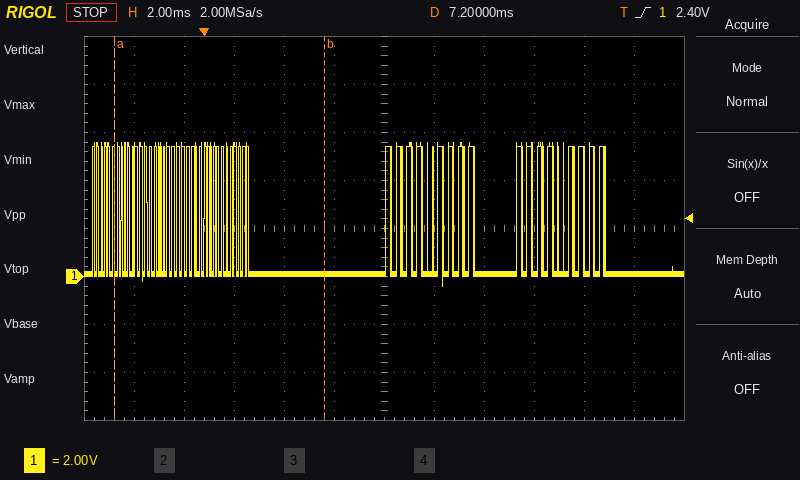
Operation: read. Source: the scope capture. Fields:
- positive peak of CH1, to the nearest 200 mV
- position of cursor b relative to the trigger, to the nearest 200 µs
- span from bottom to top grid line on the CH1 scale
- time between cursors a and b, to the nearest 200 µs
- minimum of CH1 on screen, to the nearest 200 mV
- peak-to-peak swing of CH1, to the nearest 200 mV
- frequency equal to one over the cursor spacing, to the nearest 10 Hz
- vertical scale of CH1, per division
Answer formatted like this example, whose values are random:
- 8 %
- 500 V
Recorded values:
- 5.6 V
- +4.8 ms
- 16 V
- 8.4 ms
- -400 mV
- 6.0 V
- 120 Hz
- 2 V
